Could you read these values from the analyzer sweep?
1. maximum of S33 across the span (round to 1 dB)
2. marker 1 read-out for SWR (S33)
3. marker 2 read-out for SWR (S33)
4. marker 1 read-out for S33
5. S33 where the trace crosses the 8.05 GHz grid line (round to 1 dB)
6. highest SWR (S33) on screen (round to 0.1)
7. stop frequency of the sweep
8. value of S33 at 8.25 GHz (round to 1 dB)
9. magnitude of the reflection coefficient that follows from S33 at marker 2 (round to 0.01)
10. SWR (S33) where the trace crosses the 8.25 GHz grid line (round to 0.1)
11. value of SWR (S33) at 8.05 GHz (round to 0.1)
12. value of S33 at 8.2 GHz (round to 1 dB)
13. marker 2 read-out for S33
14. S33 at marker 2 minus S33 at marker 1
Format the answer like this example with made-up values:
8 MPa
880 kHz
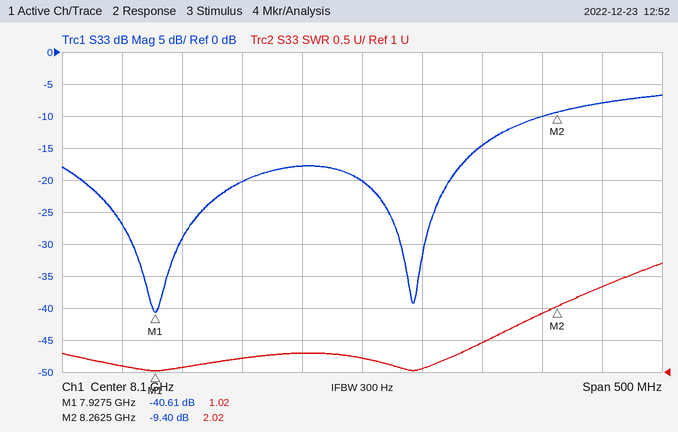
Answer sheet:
-7 dB
1.02
2.02
-40.61 dB
-18 dB
2.7
8.35 GHz
-10 dB
0.34
1.9
1.3
-15 dB
-9.40 dB
31.21 dB
